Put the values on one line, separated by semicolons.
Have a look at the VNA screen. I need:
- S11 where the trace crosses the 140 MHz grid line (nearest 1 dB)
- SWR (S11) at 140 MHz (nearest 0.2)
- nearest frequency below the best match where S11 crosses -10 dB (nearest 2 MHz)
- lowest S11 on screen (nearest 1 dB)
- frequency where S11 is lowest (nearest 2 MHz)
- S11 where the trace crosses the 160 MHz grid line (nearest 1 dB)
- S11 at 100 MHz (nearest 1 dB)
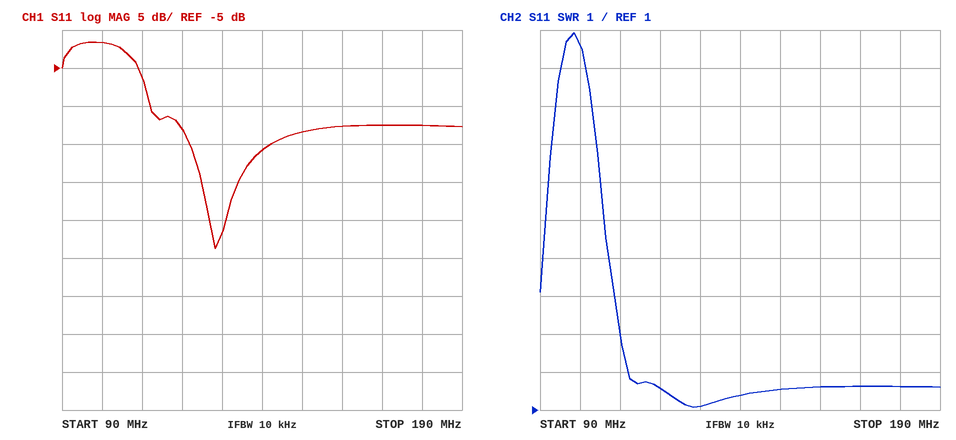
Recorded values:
-16 dB; 1.4; 112 MHz; -29 dB; 128 MHz; -13 dB; -2 dB
